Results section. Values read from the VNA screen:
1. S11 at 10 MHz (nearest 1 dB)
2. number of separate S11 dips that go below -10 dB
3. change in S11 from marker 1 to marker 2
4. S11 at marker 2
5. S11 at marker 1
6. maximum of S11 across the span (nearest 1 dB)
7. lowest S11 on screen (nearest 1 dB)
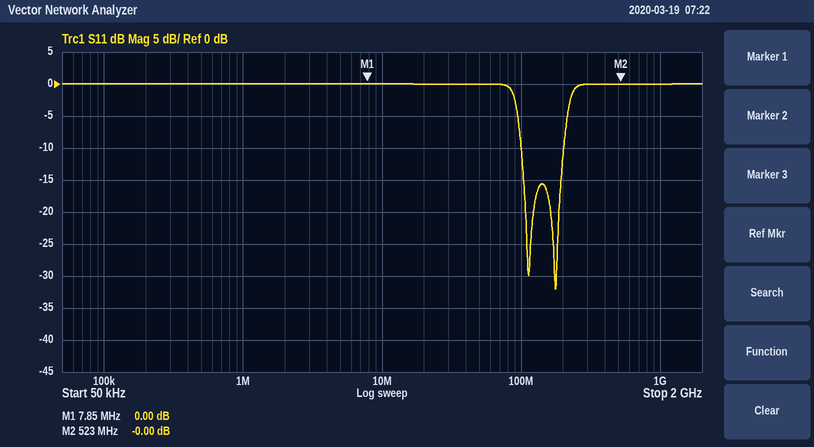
0 dB
2
0.00 dB
-0.00 dB
0.00 dB
0 dB
-32 dB
